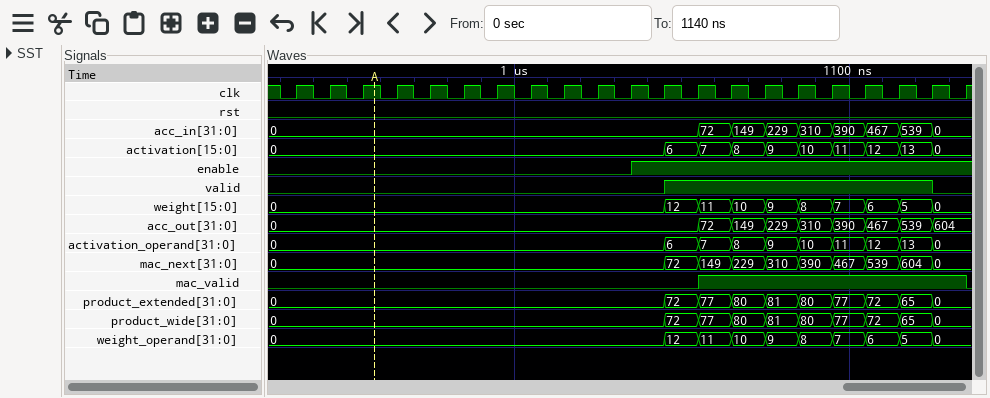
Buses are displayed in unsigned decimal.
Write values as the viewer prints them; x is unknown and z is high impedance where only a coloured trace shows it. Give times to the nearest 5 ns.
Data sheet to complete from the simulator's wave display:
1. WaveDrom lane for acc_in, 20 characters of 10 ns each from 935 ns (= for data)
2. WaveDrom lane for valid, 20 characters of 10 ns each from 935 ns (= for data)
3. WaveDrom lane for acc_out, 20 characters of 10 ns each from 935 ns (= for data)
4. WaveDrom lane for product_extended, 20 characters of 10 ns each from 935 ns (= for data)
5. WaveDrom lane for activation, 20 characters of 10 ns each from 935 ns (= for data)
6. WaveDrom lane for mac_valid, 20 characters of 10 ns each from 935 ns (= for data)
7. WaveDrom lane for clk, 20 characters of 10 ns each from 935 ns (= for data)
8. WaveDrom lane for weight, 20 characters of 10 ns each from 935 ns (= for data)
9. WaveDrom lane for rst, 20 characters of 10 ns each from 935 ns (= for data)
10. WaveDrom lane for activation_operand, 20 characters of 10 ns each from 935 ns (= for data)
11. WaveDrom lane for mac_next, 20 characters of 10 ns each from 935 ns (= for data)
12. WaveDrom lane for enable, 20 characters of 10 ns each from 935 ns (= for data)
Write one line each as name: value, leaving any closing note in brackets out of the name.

WaveDrom lane for acc_in, 20 characters of 10 ns each from 935 ns: {name: 'acc_in', wave: '=...........========', data: '0 72 149 229 310 390 467 539 0'}
WaveDrom lane for valid, 20 characters of 10 ns each from 935 ns: {name: 'valid', wave: '0..........1.......0'}
WaveDrom lane for acc_out, 20 characters of 10 ns each from 935 ns: {name: 'acc_out', wave: '=...........========', data: '0 72 149 229 310 390 467 539 604'}
WaveDrom lane for product_extended, 20 characters of 10 ns each from 935 ns: {name: 'product_extended', wave: '=..........=========', data: '0 72 77 80 81 80 77 72 65 0'}
WaveDrom lane for activation, 20 characters of 10 ns each from 935 ns: {name: 'activation', wave: '=..........=========', data: '0 6 7 8 9 10 11 12 13 0'}
WaveDrom lane for mac_valid, 20 characters of 10 ns each from 935 ns: {name: 'mac_valid', wave: '0...........1.......'}
WaveDrom lane for clk, 20 characters of 10 ns each from 935 ns: {name: 'clk', wave: 'p...................'}
WaveDrom lane for weight, 20 characters of 10 ns each from 935 ns: {name: 'weight', wave: '=..........=========', data: '0 12 11 10 9 8 7 6 5 0'}
WaveDrom lane for rst, 20 characters of 10 ns each from 935 ns: {name: 'rst', wave: '0...................'}
WaveDrom lane for activation_operand, 20 characters of 10 ns each from 935 ns: {name: 'activation_operand', wave: '=..........=========', data: '0 6 7 8 9 10 11 12 13 0'}
WaveDrom lane for mac_next, 20 characters of 10 ns each from 935 ns: {name: 'mac_next', wave: '=..........=========', data: '0 72 149 229 310 390 467 539 604 0'}
WaveDrom lane for enable, 20 characters of 10 ns each from 935 ns: {name: 'enable', wave: '0.........1.........'}
